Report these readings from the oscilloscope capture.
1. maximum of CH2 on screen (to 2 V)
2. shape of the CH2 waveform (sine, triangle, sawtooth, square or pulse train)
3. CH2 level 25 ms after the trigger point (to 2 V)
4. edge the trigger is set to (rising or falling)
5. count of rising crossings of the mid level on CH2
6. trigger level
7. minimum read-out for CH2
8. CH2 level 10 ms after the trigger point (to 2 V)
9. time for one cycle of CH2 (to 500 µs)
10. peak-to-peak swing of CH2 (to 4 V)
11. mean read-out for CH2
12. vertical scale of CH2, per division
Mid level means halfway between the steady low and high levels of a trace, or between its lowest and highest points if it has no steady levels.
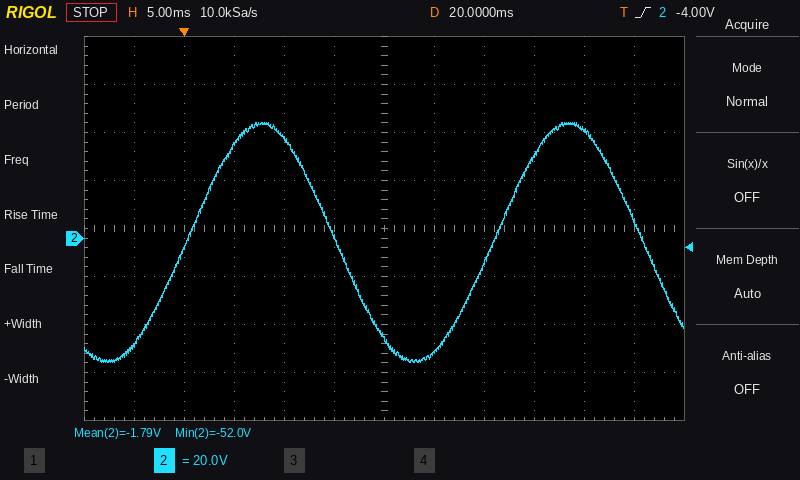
48 V
sine
-48 V
rising
2
-4.00 V
-52.0 V
42 V
30.5 ms
100 V
-1.79 V
20 V
